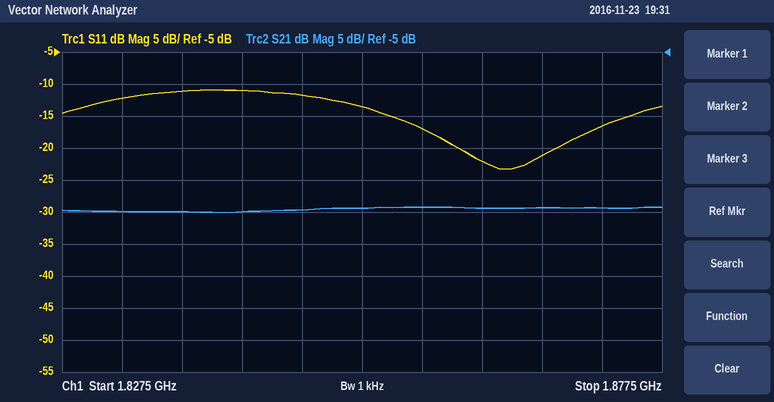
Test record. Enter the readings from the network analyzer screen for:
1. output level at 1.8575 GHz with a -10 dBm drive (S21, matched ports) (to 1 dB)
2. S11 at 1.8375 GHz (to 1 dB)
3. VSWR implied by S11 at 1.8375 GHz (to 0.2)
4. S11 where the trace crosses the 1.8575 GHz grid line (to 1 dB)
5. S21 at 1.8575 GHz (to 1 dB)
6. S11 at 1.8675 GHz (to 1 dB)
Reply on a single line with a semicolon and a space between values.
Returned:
-39 dBm; -11 dB; 1.8; -17 dB; -29 dB; -21 dB
